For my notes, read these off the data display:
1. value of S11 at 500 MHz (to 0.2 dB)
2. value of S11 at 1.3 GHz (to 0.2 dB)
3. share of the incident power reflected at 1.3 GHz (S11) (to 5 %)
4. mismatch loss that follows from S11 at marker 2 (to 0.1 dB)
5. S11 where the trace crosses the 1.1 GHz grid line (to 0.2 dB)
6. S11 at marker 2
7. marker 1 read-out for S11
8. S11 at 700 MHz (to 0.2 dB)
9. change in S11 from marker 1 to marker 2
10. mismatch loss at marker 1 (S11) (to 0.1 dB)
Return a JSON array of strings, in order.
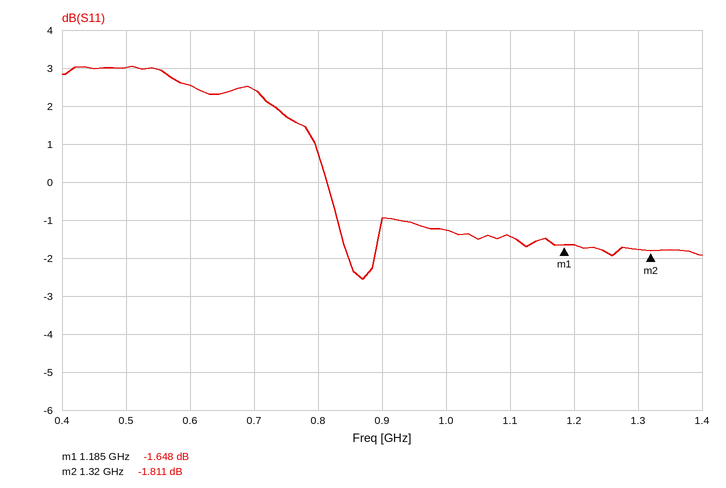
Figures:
["3.0 dB", "-1.8 dB", "65 %", "4.7 dB", "-1.4 dB", "-1.811 dB", "-1.648 dB", "2.4 dB", "-0.163 dB", "5.0 dB"]
